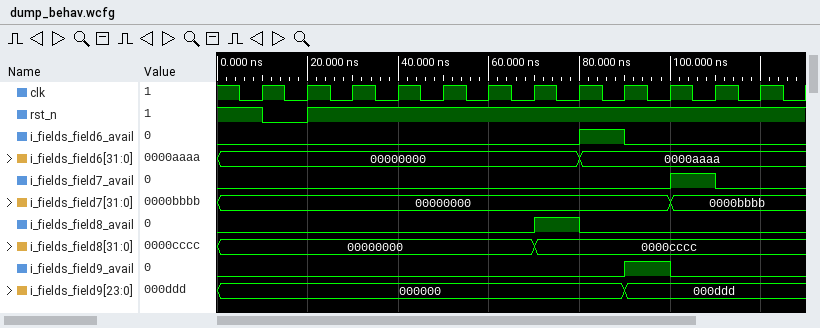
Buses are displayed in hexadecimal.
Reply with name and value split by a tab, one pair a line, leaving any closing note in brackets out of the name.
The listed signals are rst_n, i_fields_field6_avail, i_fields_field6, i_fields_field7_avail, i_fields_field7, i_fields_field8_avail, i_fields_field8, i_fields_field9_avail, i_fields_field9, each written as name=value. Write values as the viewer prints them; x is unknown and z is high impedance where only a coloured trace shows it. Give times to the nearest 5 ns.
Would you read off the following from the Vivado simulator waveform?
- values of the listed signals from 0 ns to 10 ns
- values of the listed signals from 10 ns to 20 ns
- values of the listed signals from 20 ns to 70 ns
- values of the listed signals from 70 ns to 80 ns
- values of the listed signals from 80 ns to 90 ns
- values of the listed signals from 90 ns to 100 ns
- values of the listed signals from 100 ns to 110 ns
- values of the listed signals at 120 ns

values of the listed signals from 0 ns to 10 ns	rst_n=1, i_fields_field6_avail=0, i_fields_field6=00000000, i_fields_field7_avail=0, i_fields_field7=00000000, i_fields_field8_avail=0, i_fields_field8=00000000, i_fields_field9_avail=0, i_fields_field9=000000
values of the listed signals from 10 ns to 20 ns	rst_n=0, i_fields_field6_avail=0, i_fields_field6=00000000, i_fields_field7_avail=0, i_fields_field7=00000000, i_fields_field8_avail=0, i_fields_field8=00000000, i_fields_field9_avail=0, i_fields_field9=000000
values of the listed signals from 20 ns to 70 ns	rst_n=1, i_fields_field6_avail=0, i_fields_field6=00000000, i_fields_field7_avail=0, i_fields_field7=00000000, i_fields_field8_avail=0, i_fields_field8=00000000, i_fields_field9_avail=0, i_fields_field9=000000
values of the listed signals from 70 ns to 80 ns	rst_n=1, i_fields_field6_avail=0, i_fields_field6=00000000, i_fields_field7_avail=0, i_fields_field7=00000000, i_fields_field8_avail=1, i_fields_field8=0000cccc, i_fields_field9_avail=0, i_fields_field9=000000
values of the listed signals from 80 ns to 90 ns	rst_n=1, i_fields_field6_avail=1, i_fields_field6=0000aaaa, i_fields_field7_avail=0, i_fields_field7=00000000, i_fields_field8_avail=0, i_fields_field8=0000cccc, i_fields_field9_avail=0, i_fields_field9=000000
values of the listed signals from 90 ns to 100 ns	rst_n=1, i_fields_field6_avail=0, i_fields_field6=0000aaaa, i_fields_field7_avail=0, i_fields_field7=00000000, i_fields_field8_avail=0, i_fields_field8=0000cccc, i_fields_field9_avail=1, i_fields_field9=000ddd
values of the listed signals from 100 ns to 110 ns	rst_n=1, i_fields_field6_avail=0, i_fields_field6=0000aaaa, i_fields_field7_avail=1, i_fields_field7=0000bbbb, i_fields_field8_avail=0, i_fields_field8=0000cccc, i_fields_field9_avail=0, i_fields_field9=000ddd
values of the listed signals at 120 ns	rst_n=1, i_fields_field6_avail=0, i_fields_field6=0000aaaa, i_fields_field7_avail=0, i_fields_field7=0000bbbb, i_fields_field8_avail=0, i_fields_field8=0000cccc, i_fields_field9_avail=0, i_fields_field9=000ddd
